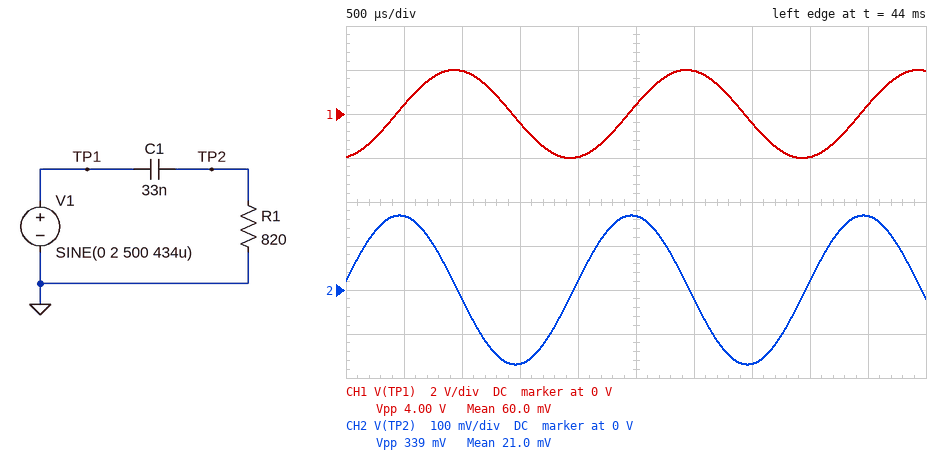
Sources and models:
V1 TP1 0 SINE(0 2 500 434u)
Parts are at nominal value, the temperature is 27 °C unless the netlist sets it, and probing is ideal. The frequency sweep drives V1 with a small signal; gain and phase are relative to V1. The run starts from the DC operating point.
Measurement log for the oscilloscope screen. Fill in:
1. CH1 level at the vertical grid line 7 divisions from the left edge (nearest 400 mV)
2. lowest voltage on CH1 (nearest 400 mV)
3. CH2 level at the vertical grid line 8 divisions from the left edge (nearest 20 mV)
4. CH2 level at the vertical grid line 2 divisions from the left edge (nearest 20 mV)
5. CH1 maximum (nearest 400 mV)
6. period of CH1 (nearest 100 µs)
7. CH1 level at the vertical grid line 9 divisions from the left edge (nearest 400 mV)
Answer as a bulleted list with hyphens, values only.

- -400 mV
- -2.0 V
- 20 mV
- -20 mV
- 2.0 V
- 2.0 ms
- 400 mV
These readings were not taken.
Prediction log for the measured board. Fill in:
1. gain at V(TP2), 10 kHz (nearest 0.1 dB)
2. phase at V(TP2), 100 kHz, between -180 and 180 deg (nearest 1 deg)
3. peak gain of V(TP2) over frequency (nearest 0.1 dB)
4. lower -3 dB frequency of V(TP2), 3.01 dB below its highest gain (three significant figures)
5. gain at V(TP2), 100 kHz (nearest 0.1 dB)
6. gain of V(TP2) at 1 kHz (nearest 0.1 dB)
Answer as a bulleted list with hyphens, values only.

- -1.3 dB
- 3 deg
- 0 dB
- 5.88 kHz
- 0 dB
- -15.5 dB
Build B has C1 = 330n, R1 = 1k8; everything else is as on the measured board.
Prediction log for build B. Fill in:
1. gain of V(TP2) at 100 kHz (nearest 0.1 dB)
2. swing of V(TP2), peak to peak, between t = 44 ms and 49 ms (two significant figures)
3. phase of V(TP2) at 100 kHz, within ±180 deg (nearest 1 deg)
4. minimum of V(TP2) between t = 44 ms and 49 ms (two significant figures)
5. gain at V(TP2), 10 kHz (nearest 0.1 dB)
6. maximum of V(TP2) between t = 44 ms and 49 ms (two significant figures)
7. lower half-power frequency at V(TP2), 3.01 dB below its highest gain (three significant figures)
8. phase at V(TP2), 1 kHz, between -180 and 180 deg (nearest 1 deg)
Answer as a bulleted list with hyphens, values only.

- 0 dB
- 3.5 V
- 0 deg
- -1.8 V
- 0 dB
- 1.8 V
- 268 Hz
- 15 deg
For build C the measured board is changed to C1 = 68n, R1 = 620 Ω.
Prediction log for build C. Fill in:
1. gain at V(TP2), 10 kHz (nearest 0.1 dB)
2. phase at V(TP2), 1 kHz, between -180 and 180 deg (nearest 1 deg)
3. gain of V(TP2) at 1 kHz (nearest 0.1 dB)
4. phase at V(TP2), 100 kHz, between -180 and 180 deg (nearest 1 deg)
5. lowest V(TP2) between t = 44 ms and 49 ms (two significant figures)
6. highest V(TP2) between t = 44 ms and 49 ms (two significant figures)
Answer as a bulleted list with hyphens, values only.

- -0.6 dB
- 75 deg
- -11.8 dB
- 2 deg
- -260 mV
- 260 mV
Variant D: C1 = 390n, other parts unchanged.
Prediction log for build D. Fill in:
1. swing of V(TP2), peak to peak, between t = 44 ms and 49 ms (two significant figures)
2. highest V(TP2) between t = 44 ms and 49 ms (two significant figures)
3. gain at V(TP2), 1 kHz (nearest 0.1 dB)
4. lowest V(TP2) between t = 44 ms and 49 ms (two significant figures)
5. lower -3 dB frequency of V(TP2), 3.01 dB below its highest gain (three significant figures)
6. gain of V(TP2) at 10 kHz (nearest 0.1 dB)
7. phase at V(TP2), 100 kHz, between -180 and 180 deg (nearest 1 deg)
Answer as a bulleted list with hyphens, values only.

- 2.8 V
- 1.4 V
- -1.0 dB
- -1.4 V
- 498 Hz
- 0 dB
- 0 deg
